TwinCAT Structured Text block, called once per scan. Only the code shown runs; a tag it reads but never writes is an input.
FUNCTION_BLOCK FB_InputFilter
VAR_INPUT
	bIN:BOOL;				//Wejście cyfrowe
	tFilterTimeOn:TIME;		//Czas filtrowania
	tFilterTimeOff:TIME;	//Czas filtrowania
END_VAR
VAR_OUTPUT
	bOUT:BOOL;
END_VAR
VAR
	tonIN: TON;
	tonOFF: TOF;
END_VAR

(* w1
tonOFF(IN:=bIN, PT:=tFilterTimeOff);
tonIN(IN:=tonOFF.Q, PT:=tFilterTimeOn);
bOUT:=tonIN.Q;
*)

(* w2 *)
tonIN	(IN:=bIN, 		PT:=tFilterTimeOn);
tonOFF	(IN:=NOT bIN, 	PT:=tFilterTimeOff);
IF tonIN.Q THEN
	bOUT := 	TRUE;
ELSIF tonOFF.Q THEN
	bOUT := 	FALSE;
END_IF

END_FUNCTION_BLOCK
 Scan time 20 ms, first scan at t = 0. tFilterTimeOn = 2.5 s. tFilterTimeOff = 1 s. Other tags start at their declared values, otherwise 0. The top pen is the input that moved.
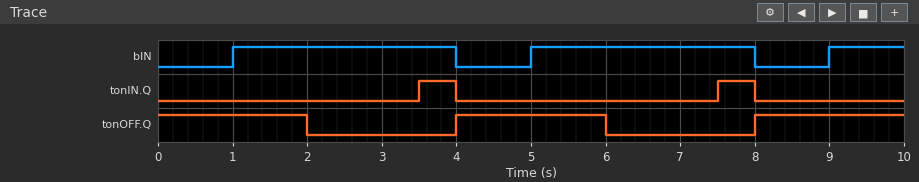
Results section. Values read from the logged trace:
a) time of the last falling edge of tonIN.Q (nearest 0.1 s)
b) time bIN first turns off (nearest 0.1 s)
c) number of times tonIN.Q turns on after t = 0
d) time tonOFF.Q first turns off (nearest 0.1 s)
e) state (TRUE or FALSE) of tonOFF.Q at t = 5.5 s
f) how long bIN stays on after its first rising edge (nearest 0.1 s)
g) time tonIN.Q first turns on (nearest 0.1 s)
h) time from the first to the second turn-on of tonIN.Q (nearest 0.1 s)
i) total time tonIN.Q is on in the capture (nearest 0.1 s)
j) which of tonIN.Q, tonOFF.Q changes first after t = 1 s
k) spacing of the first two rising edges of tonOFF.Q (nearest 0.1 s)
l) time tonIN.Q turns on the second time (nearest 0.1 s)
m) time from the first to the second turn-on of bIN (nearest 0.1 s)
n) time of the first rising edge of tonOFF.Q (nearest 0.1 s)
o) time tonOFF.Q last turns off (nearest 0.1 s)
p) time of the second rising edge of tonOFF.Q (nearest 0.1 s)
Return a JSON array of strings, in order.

["8.0 s", "4.0 s", "2", "2.0 s", "TRUE", "3.0 s", "3.5 s", "4.0 s", "1.0 s", "tonOFF.Q", "4.0 s", "7.5 s", "4.0 s", "4.0 s", "6.0 s", "8.0 s"]
